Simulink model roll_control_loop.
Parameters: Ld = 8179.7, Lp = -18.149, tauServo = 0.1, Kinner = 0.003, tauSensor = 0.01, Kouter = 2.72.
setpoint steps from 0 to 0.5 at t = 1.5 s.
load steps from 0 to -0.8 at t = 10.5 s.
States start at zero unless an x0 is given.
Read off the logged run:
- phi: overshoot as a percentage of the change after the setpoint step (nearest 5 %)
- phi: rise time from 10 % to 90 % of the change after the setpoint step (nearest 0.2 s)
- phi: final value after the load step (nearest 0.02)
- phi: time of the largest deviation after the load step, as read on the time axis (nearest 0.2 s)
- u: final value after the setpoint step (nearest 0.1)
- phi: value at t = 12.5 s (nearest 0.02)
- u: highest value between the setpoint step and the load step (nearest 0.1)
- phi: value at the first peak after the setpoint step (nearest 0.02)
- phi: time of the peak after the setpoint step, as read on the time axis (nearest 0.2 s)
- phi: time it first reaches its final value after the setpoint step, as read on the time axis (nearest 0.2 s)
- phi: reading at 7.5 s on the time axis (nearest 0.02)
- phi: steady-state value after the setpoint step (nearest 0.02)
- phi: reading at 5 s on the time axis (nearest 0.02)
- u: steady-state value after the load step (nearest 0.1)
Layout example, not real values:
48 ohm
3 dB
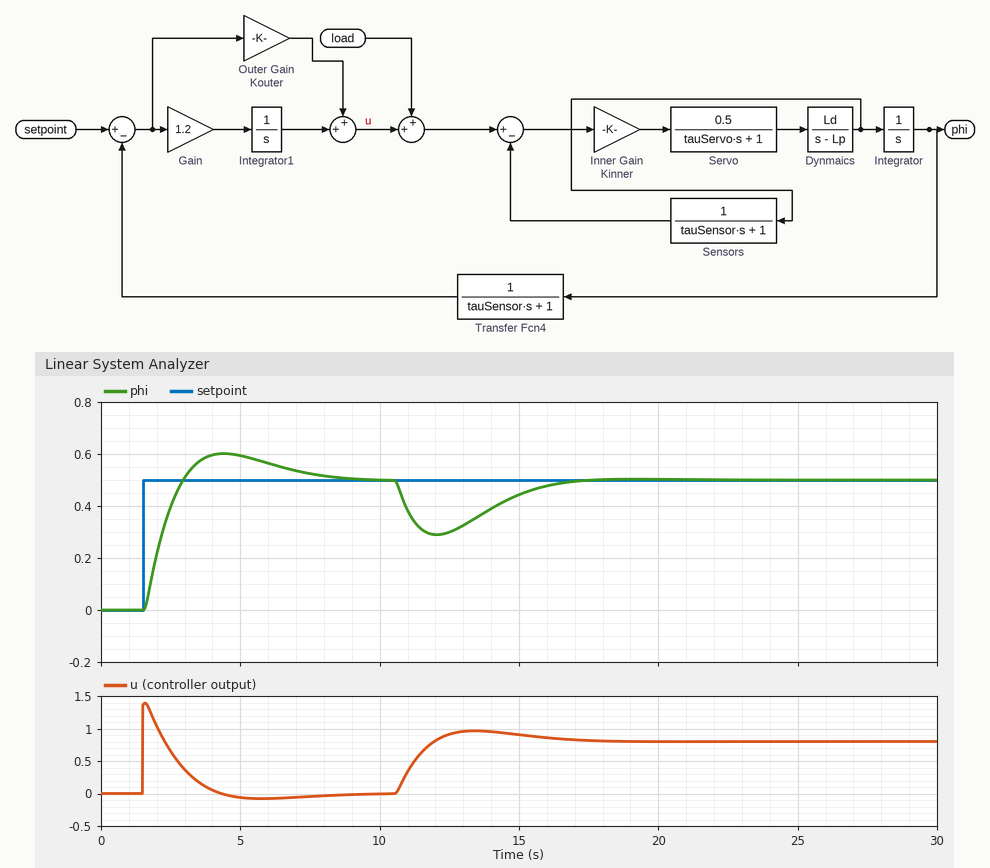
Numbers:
20 %
1.0 s
0.50
12.0 s
0.0
0.30
1.4
0.60
4.4 s
3.0 s
0.52
0.50
0.60
0.8
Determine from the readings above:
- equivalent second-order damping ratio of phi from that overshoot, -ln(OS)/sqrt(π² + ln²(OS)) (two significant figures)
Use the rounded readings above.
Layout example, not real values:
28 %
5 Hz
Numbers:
0.46
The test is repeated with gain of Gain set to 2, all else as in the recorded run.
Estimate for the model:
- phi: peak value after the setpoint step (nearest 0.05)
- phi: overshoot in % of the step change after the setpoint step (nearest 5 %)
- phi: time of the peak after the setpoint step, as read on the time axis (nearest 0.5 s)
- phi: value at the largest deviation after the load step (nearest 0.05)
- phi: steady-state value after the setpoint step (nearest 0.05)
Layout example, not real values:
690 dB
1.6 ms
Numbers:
0.65
30 %
4.0 s
0.30
0.50
